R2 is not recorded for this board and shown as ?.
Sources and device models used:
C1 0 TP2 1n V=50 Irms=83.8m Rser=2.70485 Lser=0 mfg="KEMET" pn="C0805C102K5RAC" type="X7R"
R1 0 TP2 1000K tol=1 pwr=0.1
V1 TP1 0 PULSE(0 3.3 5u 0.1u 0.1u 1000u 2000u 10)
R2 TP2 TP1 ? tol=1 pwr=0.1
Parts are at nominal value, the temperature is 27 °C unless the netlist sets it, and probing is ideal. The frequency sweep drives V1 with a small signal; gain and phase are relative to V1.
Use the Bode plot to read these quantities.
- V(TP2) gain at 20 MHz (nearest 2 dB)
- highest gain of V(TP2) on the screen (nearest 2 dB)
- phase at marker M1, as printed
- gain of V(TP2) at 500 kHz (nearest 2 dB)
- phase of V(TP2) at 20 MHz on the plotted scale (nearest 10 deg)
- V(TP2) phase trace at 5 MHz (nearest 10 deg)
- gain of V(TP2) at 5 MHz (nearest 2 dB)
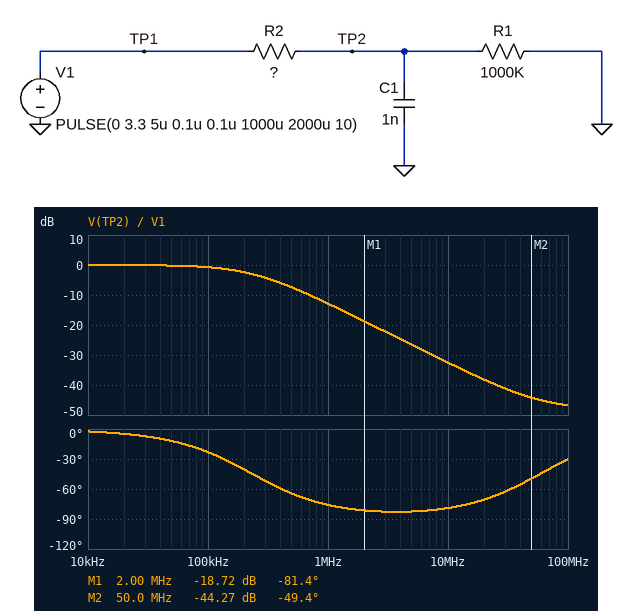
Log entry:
-38 dB
0 dB
-81.4 deg
-8 dB
-70 deg
-80 deg
-26 dB
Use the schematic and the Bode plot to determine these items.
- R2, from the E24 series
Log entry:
680 Ω
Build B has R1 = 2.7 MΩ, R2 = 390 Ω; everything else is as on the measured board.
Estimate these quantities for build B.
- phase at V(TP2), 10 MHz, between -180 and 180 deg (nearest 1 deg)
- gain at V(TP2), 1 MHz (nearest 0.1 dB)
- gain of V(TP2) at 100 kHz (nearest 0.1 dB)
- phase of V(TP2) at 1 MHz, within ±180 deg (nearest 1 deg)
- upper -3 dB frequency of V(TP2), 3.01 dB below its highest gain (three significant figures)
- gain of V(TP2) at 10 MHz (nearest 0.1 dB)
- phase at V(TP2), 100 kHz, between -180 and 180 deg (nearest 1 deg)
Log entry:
-78 deg
-8.5 dB
-0.3 dB
-67 deg
405 kHz
-27.7 dB
-14 deg
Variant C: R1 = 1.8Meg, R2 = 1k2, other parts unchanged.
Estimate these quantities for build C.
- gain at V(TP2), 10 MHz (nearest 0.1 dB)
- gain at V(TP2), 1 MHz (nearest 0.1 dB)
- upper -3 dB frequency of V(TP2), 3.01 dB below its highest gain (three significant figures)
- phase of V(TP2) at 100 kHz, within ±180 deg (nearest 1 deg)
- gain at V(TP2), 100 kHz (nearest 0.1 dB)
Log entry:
-37.4 dB
-17.6 dB
132 kHz
-37 deg
-2.0 dB
